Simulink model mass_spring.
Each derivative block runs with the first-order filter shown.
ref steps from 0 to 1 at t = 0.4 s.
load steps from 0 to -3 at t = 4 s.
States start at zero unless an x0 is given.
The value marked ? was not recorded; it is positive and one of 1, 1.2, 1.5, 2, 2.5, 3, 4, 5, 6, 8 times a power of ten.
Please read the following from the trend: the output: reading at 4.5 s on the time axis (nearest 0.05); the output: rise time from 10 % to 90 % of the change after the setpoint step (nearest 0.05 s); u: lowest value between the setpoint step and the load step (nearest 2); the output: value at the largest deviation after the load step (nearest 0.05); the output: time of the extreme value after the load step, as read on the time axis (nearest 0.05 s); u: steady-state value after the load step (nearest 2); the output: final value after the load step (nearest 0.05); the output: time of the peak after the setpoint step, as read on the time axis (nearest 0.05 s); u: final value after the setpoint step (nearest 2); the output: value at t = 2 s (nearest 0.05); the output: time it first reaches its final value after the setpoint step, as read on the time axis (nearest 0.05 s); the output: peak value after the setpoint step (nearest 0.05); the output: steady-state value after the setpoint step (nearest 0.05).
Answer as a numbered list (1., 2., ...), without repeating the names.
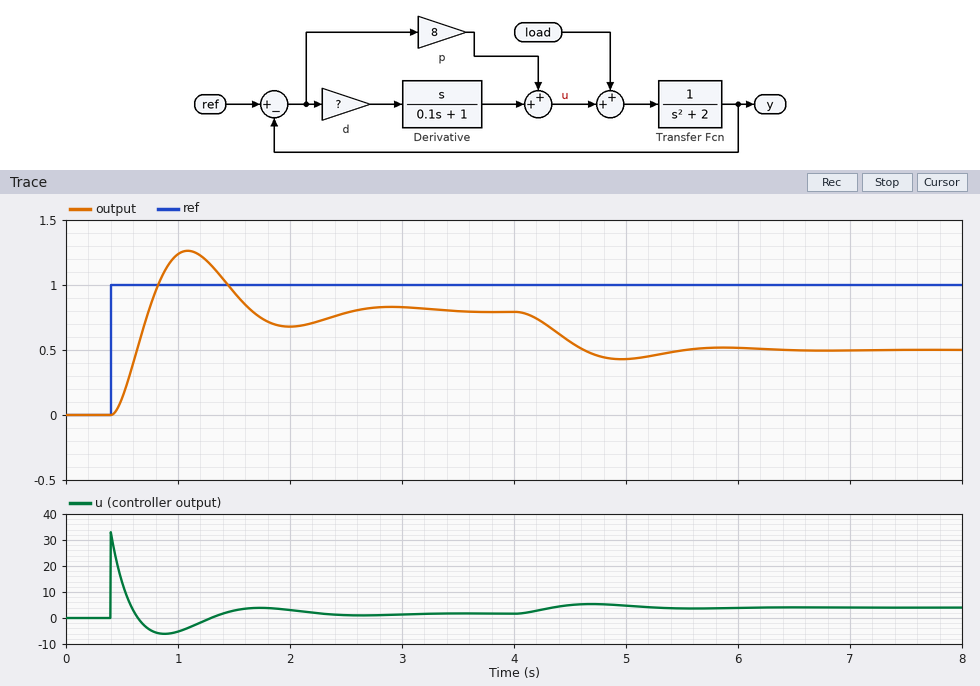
1. 0.55
2. 0.25 s
3. -6
4. 0.45
5. 4.95 s
6. 4
7. 0.50
8. 1.10 s
9. 2
10. 0.70
11. 0.75 s
12. 1.25
13. 0.80
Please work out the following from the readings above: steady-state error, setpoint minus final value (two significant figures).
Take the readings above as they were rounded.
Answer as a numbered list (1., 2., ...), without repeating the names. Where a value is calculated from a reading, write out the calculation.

1. 1 - 0.8 = 0.20
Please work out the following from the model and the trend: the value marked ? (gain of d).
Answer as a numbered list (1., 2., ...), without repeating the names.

1. 2.5
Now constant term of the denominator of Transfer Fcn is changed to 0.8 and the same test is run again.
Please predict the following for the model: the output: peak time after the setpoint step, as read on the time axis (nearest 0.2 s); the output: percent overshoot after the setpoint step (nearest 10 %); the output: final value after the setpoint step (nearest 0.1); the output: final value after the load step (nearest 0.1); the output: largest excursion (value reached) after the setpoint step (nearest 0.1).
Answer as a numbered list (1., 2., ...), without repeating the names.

1. 1.2 s
2. 50 %
3. 0.9
4. 0.6
5. 1.4
